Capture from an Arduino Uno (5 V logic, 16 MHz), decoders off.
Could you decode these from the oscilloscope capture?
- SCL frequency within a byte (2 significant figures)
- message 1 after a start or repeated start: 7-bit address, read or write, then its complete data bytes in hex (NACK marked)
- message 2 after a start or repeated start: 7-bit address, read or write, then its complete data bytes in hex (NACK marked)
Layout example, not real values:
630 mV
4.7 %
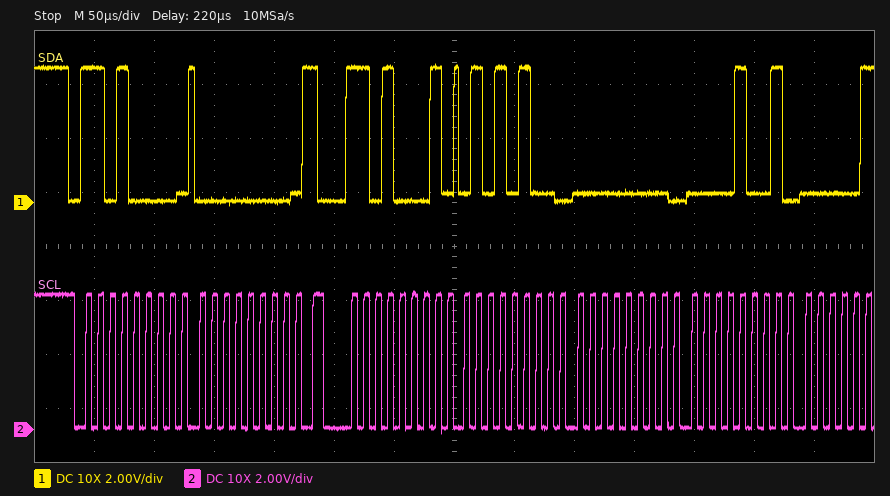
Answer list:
100 kHz
0x68 write: 00
0x68 read: 54 00 09
